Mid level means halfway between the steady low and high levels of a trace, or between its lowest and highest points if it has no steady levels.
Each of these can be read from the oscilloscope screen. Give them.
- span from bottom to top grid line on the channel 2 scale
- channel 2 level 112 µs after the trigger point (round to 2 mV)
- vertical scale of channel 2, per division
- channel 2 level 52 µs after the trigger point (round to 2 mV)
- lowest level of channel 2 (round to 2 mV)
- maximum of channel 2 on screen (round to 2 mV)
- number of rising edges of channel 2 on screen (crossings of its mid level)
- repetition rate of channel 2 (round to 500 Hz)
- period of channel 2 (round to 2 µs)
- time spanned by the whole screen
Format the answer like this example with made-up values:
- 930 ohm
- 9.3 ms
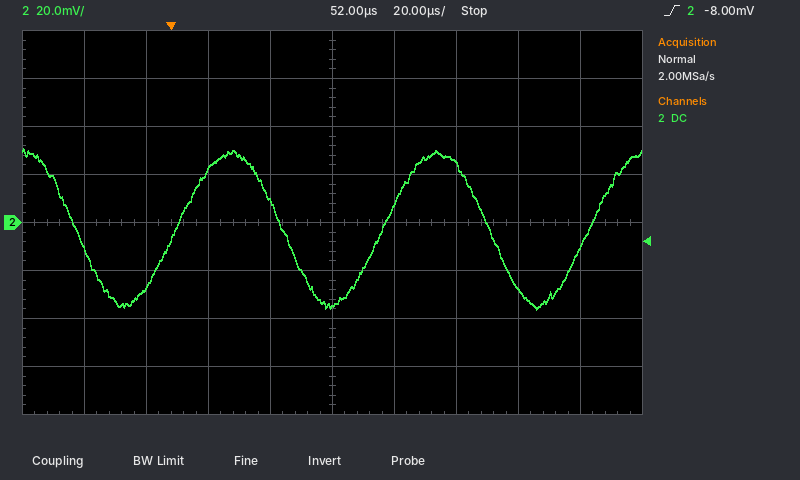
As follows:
- 160 mV
- -28 mV
- 20 mV
- -34 mV
- -36 mV
- 30 mV
- 3
- 15.0 kHz
- 66 µs
- 200 µs
